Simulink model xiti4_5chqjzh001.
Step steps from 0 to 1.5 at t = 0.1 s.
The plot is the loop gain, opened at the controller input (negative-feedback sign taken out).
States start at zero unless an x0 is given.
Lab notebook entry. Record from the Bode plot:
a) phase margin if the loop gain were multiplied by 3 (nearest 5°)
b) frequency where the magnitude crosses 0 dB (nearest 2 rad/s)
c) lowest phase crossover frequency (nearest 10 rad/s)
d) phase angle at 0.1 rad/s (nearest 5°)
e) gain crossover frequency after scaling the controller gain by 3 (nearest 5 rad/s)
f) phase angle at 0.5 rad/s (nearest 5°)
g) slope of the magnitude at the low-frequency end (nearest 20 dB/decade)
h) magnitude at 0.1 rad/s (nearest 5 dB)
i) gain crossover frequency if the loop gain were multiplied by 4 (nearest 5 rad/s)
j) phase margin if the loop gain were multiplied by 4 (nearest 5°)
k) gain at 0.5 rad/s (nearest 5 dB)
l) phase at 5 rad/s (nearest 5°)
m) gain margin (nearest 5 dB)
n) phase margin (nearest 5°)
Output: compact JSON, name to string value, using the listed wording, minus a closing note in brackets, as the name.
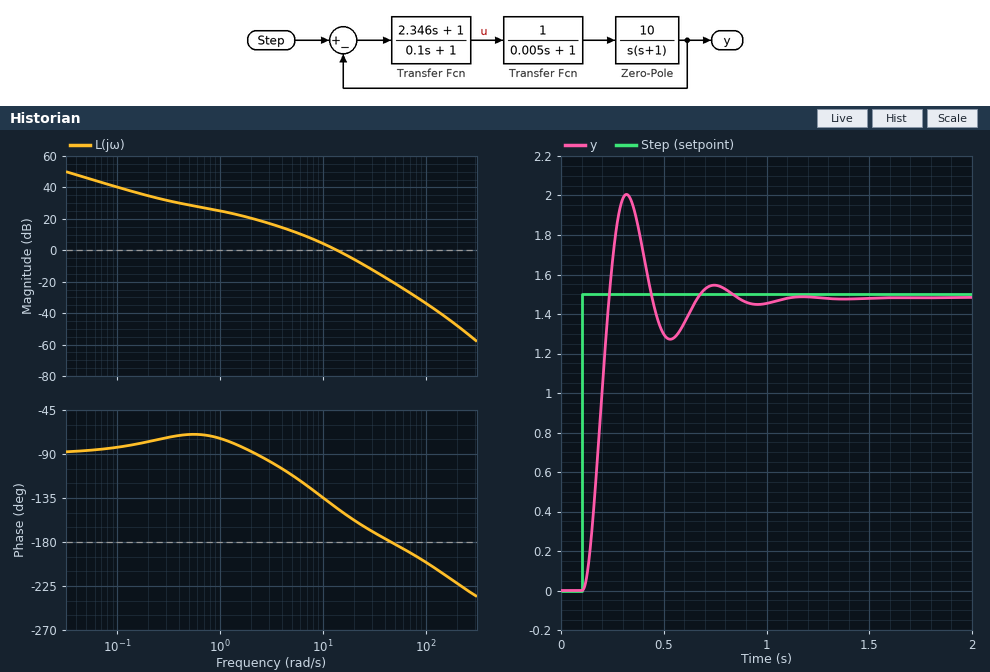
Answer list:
{"phase margin if the loop gain were multiplied by 3": "15°", "frequency where the magnitude crosses 0 dB": "14 rad/s", "lowest phase crossover frequency": "50 rad/s", "phase angle at 0.1 rad/s": "-85°", "gain crossover frequency after scaling the controller gain by 3": "25 rad/s", "phase angle at 0.5 rad/s": "-70°", "slope of the magnitude at the low-frequency end": "-20 dB/decade", "magnitude at 0.1 rad/s": "40 dB", "gain crossover frequency if the loop gain were multiplied by 4": "30 rad/s", "phase margin if the loop gain were multiplied by 4": "10°", "gain at 0.5 rad/s": "30 dB", "phase at 5 rad/s": "-110°", "gain margin": "20 dB", "phase margin": "35°"}
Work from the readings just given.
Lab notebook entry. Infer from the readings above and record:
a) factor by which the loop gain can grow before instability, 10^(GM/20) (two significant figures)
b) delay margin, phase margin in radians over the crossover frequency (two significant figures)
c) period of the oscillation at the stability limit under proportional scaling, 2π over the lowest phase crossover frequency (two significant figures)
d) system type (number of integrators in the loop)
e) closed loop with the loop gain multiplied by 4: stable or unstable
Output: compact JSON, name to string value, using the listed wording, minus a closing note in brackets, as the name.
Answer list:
{"factor by which the loop gain can grow before instability, 10^(GM/20)": "10", "delay margin, phase margin in radians over the crossover frequency": "0.044 s", "period of the oscillation at the stability limit under proportional scaling, 2π over the lowest phase crossover frequency": "0.13 s", "system type": "1", "closed loop with the loop gain multiplied by 4: stable or unstable": "stable"}
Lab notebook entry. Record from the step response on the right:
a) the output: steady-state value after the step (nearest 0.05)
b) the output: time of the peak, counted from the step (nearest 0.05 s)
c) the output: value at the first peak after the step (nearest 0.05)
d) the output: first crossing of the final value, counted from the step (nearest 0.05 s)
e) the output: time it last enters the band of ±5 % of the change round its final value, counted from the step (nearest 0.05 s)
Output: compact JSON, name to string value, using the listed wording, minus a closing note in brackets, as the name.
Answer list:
{"the output: steady-state value after the step": "1.50", "the output: time of the peak, counted from the step": "0.20 s", "the output: value at the first peak after the step": "2.00", "the output: first crossing of the final value, counted from the step": "0.15 s", "the output: time it last enters the band of ±5 % of the change round its final value, counted from the step": "0.55 s"}
